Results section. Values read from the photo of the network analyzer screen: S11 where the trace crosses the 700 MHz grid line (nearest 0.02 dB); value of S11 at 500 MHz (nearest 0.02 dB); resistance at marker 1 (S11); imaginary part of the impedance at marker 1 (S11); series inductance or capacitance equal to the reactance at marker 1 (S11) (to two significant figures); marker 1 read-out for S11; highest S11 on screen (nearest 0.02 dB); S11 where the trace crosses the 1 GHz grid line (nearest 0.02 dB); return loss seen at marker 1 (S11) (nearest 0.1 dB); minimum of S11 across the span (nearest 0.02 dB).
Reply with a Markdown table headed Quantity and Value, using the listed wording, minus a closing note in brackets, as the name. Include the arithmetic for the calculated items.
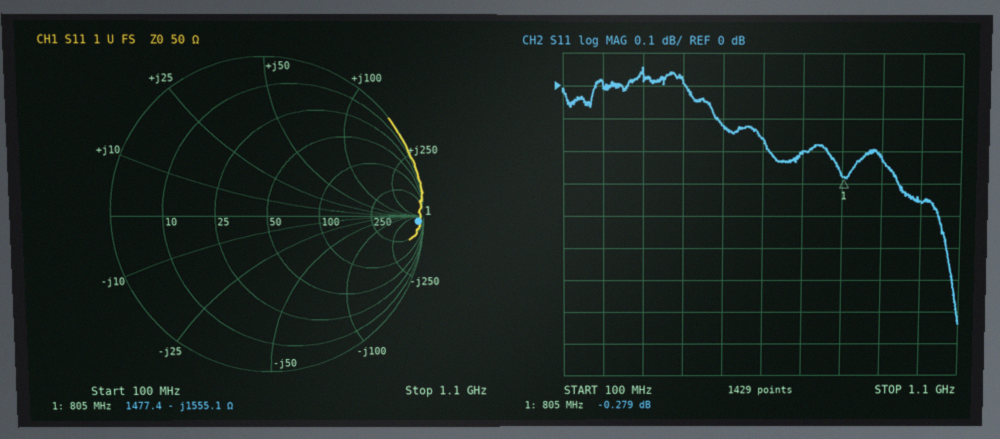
| Quantity | Value |
|---|---|
| S11 where the trace crosses the 700 MHz grid line | -0.20 dB |
| value of S11 at 500 MHz | -0.12 dB |
| resistance at marker 1 | 1477.4 Ω |
| imaginary part of the impedance at marker 1 | -1555.1 Ω |
| series inductance or capacitance equal to the reactance at marker 1 (S11) | C = 1/(2π × 805 MHz × 1555.1 Ω) ≈ 127 fF, so 130 fF to two significant figures |
| marker 1 read-out for S11 | -0.279 dB |
| highest S11 on screen | 0.06 dB |
| S11 where the trace crosses the 1 GHz grid line | -0.36 dB |
| return loss seen at marker 1 (S11) | 0.3 dB |
| minimum of S11 across the span | -0.74 dB |
